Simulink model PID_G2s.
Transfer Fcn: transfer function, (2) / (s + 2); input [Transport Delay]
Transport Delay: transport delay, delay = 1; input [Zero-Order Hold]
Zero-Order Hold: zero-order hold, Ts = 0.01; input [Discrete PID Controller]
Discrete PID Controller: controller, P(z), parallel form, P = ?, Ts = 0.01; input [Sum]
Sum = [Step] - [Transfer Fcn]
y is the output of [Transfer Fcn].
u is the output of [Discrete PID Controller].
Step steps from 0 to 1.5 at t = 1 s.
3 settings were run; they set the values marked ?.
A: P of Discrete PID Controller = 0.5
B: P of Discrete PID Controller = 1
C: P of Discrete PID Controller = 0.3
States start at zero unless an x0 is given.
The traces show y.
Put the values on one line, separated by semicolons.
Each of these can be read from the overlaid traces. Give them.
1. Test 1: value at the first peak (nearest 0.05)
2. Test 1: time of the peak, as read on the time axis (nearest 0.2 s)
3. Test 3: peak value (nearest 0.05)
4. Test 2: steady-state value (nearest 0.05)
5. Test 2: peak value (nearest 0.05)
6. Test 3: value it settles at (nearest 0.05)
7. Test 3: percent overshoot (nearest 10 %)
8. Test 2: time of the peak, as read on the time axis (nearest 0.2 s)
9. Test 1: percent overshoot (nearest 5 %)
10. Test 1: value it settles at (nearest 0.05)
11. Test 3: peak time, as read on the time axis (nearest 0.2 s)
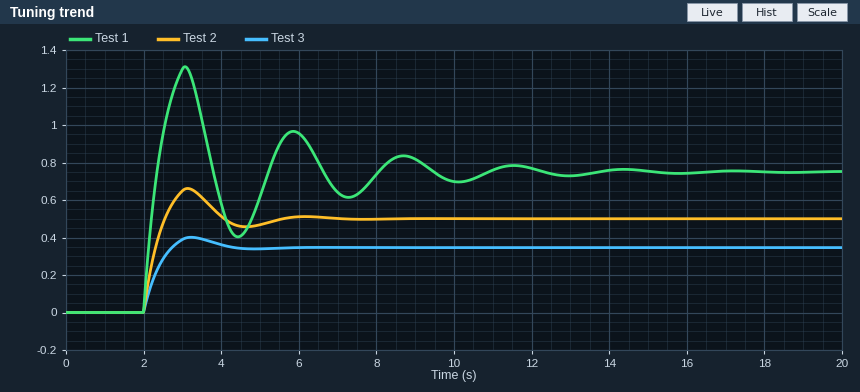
1.30; 3.0 s; 0.40; 0.50; 0.65; 0.35; 20 %; 3.2 s; 75 %; 0.75; 3.2 s
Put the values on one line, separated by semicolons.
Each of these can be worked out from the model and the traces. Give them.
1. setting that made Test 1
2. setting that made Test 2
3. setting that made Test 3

B; A; C
